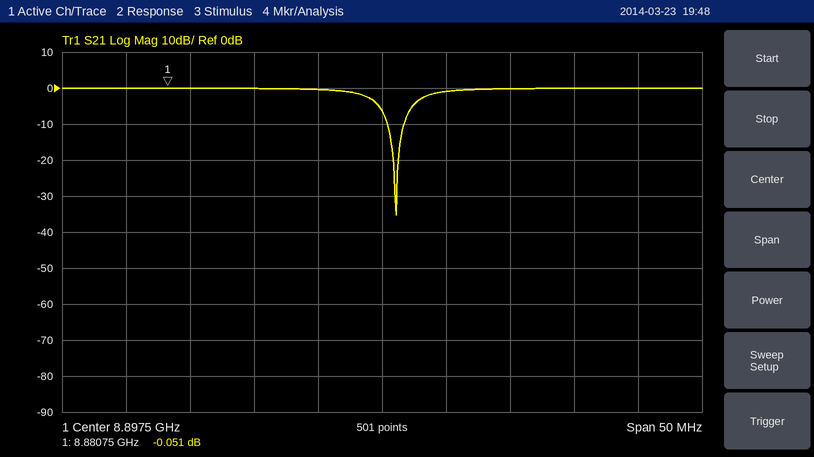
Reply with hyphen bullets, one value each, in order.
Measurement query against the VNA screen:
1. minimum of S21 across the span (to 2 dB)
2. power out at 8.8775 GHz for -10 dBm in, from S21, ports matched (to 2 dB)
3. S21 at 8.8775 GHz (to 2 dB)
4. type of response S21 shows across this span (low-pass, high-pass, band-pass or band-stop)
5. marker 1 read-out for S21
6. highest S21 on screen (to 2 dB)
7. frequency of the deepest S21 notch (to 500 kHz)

- -36 dB
- -10 dBm
- 0 dB
- band-stop
- -0.051 dB
- 0 dB
- 8.8985 GHz
